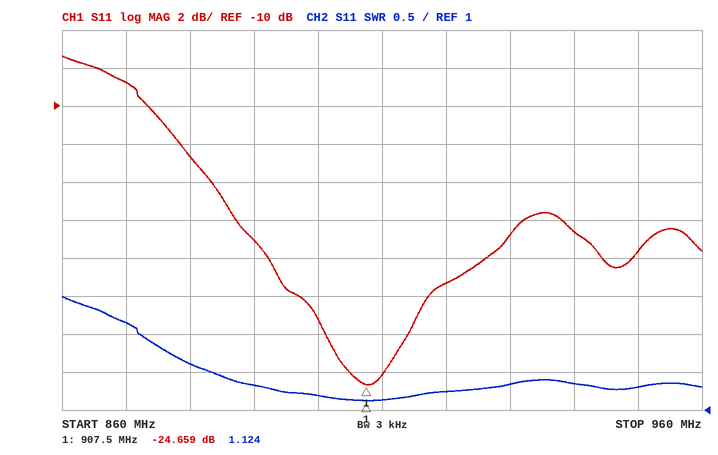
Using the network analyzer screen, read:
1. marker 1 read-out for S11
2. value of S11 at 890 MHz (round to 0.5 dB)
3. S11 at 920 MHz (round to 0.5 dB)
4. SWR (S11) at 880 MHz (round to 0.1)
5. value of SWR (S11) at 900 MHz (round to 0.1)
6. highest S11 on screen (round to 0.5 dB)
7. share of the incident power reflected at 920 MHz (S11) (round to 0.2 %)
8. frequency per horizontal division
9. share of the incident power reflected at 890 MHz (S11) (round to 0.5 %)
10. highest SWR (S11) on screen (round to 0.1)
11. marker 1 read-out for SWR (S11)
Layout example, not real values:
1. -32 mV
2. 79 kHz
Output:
1. -24.659 dB
2. -17.0 dB
3. -19.5 dB
4. 1.6
5. 1.2
6. -7.5 dB
7. 1.2 %
8. 10 MHz
9. 2.0 %
10. 2.5
11. 1.124
